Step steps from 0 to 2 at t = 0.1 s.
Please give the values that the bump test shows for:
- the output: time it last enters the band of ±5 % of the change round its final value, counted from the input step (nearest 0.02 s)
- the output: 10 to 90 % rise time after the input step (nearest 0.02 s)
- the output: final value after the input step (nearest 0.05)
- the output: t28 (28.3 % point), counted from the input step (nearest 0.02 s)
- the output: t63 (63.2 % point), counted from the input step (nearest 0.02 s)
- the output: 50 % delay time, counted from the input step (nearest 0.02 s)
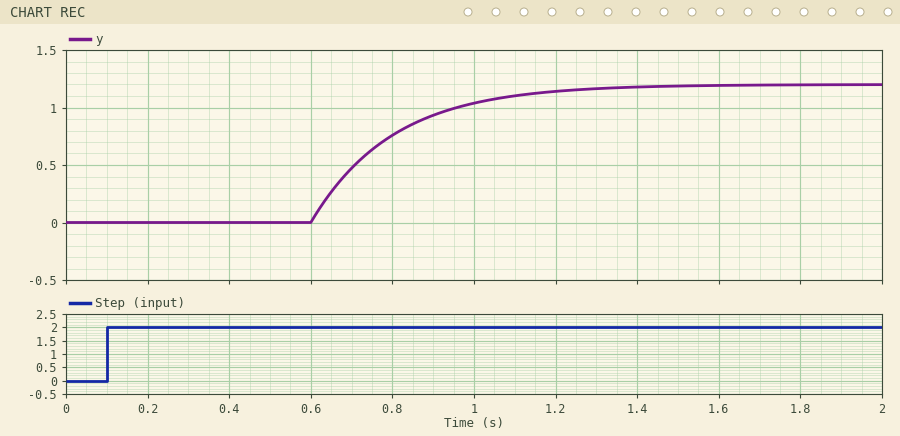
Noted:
1.10 s
0.44 s
1.20
0.56 s
0.70 s
0.64 s
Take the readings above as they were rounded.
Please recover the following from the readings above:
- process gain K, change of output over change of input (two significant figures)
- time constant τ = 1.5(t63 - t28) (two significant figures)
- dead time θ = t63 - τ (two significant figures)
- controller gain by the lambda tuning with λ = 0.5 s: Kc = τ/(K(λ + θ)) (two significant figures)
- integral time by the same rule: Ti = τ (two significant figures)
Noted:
0.60
0.21 s
0.49 s
0.35
0.21 s
